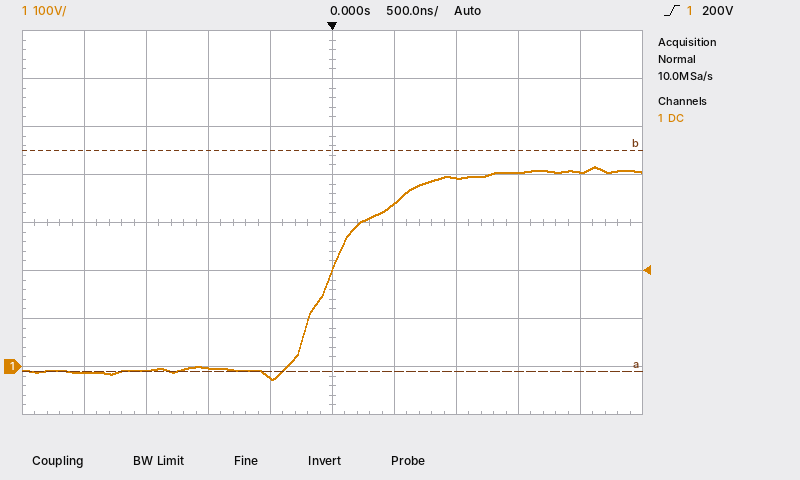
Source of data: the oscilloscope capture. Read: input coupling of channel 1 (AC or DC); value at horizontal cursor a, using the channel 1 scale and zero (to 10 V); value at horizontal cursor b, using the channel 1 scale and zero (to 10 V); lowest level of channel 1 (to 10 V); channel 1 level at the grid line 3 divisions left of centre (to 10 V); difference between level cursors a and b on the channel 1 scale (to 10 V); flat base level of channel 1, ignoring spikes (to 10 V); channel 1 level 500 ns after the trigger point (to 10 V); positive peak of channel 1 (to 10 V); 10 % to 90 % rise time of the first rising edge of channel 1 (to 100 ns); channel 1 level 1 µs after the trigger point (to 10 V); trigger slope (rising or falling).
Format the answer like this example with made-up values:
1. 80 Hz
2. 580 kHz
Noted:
1. DC
2. -10 V
3. 450 V
4. -30 V
5. -10 V
6. 460 V
7. -10 V
8. 340 V
9. 420 V
10. 900 ns
11. 390 V
12. rising
